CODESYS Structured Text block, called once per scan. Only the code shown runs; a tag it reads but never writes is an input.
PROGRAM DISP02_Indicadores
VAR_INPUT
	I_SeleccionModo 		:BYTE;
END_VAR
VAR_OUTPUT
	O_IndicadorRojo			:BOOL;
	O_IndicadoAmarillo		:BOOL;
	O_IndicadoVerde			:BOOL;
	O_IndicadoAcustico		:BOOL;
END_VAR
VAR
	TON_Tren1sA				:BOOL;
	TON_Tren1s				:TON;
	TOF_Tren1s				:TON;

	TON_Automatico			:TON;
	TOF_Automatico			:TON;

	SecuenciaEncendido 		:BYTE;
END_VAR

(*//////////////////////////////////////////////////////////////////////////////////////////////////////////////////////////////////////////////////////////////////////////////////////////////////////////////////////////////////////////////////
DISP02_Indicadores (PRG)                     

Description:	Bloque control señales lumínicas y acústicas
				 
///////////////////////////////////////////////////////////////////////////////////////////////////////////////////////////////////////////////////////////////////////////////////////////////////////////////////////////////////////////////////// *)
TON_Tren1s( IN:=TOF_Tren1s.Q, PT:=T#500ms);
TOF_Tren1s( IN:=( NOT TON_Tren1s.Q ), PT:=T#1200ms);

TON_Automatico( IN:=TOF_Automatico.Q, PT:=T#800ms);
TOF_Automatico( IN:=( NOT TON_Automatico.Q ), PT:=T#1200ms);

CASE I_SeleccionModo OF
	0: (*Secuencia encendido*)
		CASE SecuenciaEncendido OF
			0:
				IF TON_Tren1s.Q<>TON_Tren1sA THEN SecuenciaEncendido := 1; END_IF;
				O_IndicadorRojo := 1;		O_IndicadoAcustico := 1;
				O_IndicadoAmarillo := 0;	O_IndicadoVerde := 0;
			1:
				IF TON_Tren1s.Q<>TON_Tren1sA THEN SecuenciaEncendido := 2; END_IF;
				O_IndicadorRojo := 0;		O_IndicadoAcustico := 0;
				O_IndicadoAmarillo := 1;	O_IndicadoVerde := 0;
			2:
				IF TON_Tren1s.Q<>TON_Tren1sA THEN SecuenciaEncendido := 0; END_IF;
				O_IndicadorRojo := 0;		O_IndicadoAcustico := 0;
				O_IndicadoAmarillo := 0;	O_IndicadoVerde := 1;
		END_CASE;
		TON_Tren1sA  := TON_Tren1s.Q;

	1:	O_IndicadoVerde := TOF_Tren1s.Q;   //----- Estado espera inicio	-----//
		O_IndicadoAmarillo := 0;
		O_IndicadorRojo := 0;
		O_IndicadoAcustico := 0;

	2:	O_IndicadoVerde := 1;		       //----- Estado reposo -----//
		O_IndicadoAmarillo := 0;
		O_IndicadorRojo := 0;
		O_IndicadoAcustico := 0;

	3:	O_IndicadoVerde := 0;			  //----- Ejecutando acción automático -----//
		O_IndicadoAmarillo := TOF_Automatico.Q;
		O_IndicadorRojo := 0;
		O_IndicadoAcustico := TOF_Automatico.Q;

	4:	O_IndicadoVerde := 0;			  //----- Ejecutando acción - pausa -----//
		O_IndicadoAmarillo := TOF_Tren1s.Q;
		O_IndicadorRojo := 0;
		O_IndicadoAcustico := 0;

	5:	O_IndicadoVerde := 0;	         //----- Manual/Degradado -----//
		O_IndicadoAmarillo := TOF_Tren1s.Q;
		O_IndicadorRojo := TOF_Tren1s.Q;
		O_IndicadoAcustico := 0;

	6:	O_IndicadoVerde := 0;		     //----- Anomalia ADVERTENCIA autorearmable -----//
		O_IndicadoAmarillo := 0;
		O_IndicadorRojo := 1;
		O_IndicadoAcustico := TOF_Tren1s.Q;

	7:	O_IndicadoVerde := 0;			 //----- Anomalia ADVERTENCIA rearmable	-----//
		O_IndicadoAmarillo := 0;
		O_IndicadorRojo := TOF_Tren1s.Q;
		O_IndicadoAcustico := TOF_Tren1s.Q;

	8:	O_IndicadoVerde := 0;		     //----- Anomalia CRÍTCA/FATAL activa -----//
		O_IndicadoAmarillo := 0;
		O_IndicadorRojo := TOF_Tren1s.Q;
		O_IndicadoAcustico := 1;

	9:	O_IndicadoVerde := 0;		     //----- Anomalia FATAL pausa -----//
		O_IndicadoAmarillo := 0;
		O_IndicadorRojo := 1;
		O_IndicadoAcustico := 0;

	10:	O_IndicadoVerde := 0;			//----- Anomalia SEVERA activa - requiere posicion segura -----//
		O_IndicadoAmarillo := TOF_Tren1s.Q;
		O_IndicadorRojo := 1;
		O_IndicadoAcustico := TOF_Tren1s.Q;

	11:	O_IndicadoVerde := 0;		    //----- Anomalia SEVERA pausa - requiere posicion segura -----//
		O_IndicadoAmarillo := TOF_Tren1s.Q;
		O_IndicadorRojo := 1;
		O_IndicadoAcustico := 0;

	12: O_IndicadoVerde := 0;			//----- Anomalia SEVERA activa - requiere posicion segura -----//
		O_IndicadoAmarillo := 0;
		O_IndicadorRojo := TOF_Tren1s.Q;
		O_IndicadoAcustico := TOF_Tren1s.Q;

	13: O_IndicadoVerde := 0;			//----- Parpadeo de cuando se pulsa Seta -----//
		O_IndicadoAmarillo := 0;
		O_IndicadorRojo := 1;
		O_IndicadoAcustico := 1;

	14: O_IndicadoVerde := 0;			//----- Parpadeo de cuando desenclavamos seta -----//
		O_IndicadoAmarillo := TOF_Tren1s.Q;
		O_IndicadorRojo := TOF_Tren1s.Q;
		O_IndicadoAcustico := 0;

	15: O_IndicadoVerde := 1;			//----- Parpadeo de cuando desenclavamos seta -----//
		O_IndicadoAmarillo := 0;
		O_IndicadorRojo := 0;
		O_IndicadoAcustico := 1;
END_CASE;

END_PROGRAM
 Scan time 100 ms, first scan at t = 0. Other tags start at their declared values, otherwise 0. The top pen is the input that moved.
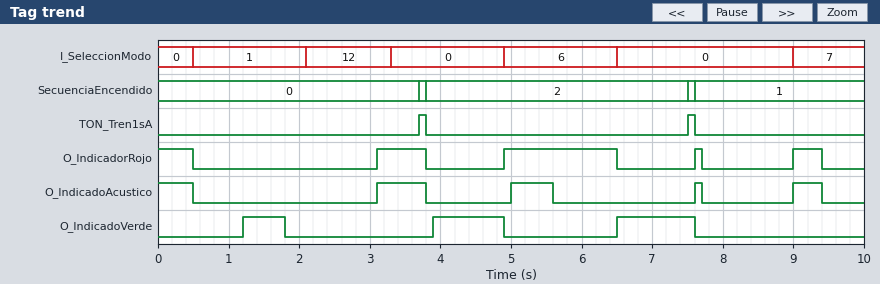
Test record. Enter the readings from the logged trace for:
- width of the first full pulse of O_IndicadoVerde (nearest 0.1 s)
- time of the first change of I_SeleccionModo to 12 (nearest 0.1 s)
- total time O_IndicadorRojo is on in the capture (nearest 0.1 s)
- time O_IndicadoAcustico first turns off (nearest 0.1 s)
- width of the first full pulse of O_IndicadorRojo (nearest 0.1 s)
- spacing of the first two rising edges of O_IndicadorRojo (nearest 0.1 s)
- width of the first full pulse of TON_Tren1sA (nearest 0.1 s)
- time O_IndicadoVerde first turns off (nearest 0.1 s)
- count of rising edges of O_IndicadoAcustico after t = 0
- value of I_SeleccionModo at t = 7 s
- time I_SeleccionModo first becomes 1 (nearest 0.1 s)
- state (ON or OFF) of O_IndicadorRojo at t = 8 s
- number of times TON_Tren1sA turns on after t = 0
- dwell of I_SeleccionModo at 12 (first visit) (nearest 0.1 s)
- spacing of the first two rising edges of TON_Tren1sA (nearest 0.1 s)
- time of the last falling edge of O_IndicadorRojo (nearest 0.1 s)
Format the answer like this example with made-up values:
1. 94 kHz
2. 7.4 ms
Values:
1. 0.6 s
2. 2.1 s
3. 3.3 s
4. 0.5 s
5. 0.7 s
6. 1.8 s
7. 0.1 s
8. 1.8 s
9. 4
10. 0
11. 0.5 s
12. OFF
13. 2
14. 1.2 s
15. 3.8 s
16. 9.4 s
